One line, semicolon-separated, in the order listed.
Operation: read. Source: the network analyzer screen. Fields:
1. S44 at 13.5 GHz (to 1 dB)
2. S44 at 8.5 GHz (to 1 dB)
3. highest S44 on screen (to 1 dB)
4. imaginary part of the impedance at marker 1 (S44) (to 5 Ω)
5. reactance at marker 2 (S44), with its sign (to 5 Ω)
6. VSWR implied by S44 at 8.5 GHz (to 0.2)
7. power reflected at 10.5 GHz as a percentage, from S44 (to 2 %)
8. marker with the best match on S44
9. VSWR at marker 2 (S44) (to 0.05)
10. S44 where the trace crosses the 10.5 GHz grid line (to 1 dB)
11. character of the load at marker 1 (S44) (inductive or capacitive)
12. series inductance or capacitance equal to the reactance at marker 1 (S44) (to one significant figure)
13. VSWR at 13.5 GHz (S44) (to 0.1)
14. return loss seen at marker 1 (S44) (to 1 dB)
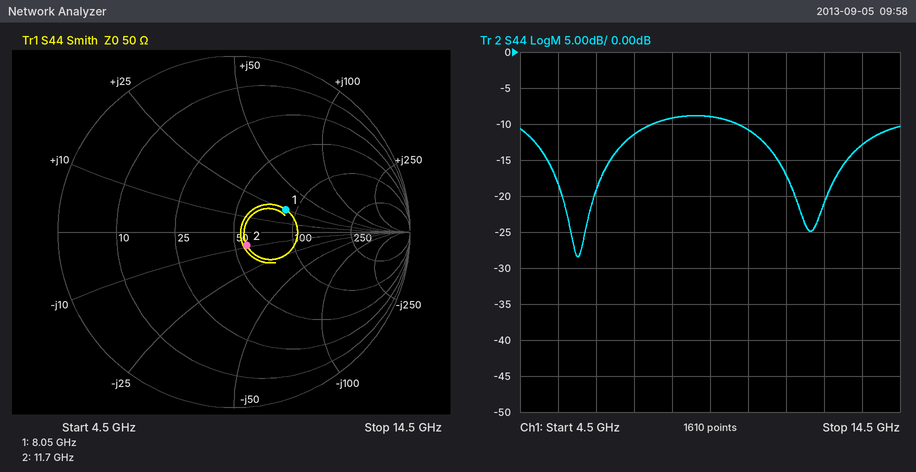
-13 dB; -9 dB; -9 dB; +25 Ω; -10 Ω; 2.0; 8 %; marker 2; 1.25; -11 dB; inductive; 500 pH; 1.6; 10 dB
